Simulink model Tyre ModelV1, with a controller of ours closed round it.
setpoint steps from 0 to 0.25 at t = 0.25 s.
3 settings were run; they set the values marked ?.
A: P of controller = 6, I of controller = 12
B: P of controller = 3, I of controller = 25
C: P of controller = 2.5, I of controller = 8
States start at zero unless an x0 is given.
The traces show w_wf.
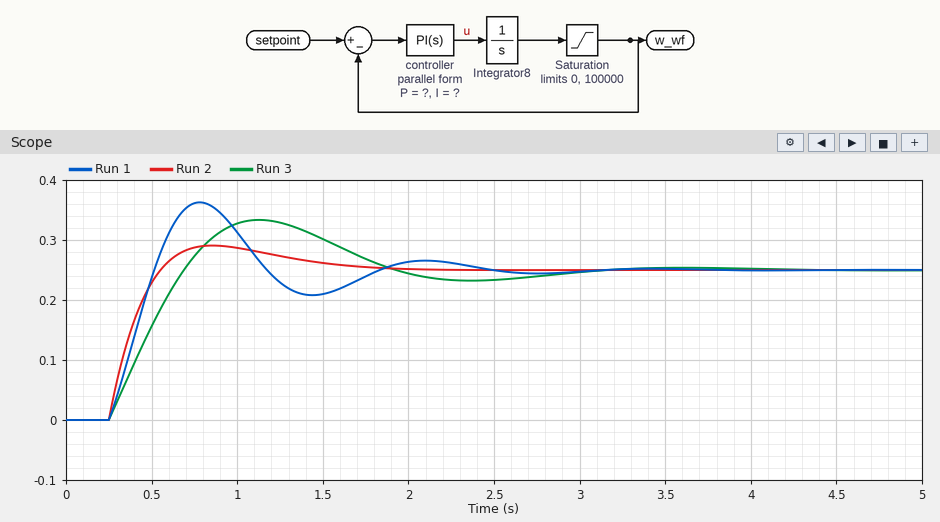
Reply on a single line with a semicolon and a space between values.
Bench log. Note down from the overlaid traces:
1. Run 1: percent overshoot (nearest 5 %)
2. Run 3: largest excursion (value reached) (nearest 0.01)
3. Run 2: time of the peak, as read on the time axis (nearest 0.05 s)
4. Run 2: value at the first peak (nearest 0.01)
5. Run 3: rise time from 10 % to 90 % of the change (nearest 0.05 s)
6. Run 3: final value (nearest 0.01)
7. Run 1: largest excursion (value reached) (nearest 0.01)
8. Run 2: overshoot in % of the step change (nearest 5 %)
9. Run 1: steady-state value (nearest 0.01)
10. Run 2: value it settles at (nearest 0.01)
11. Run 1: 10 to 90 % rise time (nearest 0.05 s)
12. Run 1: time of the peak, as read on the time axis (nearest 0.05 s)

45 %; 0.33; 0.85 s; 0.29; 0.35 s; 0.25; 0.36; 15 %; 0.25; 0.25; 0.20 s; 0.80 s
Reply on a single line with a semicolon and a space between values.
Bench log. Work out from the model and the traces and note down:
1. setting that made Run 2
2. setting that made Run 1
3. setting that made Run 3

A; B; C
